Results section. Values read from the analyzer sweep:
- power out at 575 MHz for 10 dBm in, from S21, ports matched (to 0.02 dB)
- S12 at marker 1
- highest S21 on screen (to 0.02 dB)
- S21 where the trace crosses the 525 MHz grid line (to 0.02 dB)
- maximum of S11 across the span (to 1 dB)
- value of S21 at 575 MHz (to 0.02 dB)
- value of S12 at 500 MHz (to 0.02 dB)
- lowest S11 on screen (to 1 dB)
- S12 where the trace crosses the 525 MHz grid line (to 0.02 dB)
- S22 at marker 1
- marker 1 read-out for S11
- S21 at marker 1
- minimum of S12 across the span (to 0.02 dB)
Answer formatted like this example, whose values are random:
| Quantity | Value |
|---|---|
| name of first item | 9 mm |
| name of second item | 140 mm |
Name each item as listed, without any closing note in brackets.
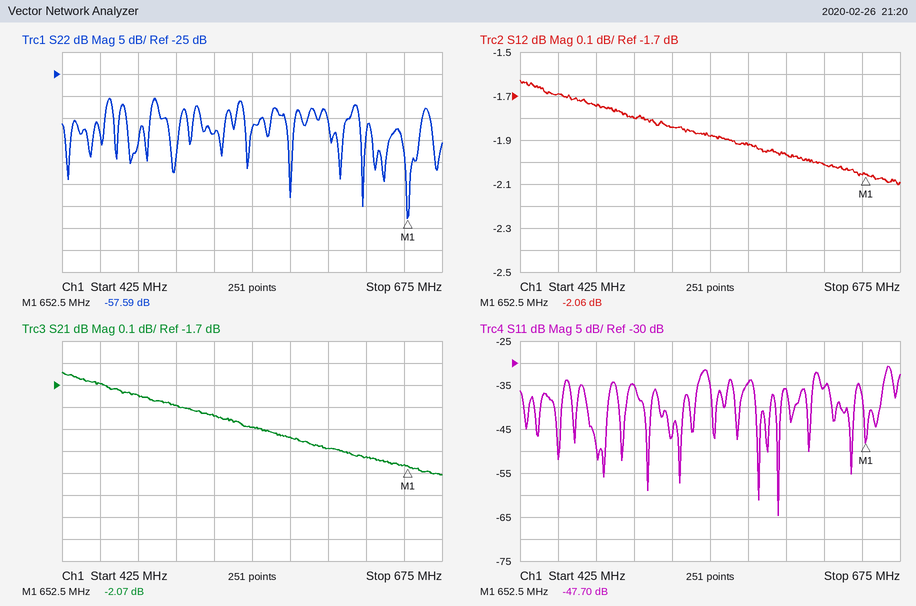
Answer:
| Quantity | Value |
|---|---|
| power out at 575 MHz for 10 dBm in, from S21, ports matched | 8.06 dBm |
| S12 at marker 1 | -2.06 dB |
| highest S21 on screen | -1.64 dB |
| S21 where the trace crosses the 525 MHz grid line | -1.84 dB |
| maximum of S11 across the span | -31 dB |
| value of S21 at 575 MHz | -1.94 dB |
| value of S12 at 500 MHz | -1.80 dB |
| lowest S11 on screen | -65 dB |
| S12 where the trace crosses the 525 MHz grid line | -1.84 dB |
| S22 at marker 1 | -57.59 dB |
| marker 1 read-out for S11 | -47.70 dB |
| S21 at marker 1 | -2.07 dB |
| minimum of S12 across the span | -2.10 dB |
